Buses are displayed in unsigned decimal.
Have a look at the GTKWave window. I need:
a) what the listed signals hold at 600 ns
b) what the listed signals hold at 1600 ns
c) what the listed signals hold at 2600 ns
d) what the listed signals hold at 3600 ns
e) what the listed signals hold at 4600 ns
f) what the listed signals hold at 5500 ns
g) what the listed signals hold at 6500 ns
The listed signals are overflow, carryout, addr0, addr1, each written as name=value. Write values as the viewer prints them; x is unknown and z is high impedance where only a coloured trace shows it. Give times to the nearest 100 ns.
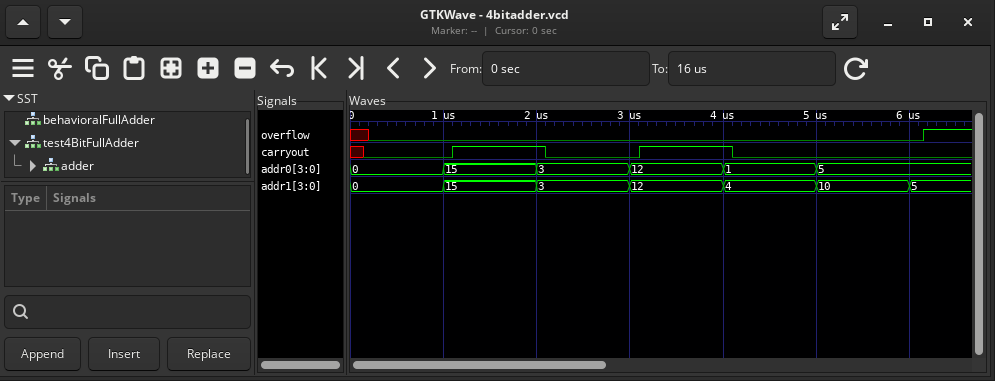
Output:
overflow=0, carryout=0, addr0=0, addr1=0
overflow=0, carryout=1, addr0=15, addr1=15
overflow=0, carryout=0, addr0=3, addr1=3
overflow=0, carryout=1, addr0=12, addr1=12
overflow=0, carryout=0, addr0=1, addr1=4
overflow=0, carryout=0, addr0=5, addr1=10
overflow=1, carryout=0, addr0=5, addr1=5
